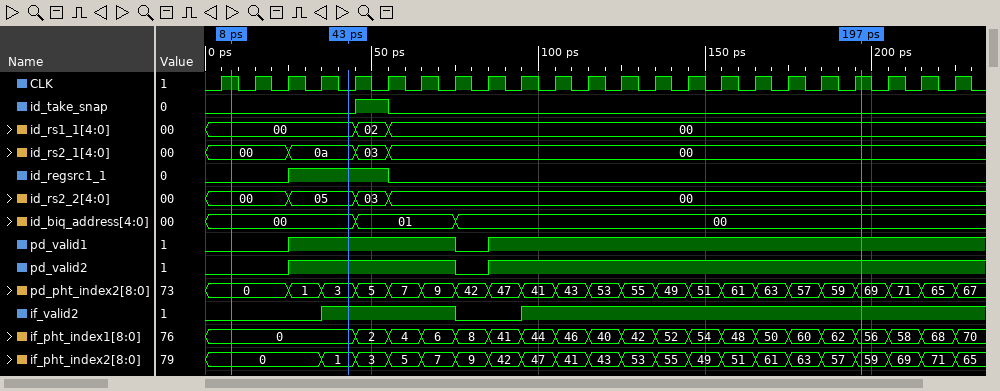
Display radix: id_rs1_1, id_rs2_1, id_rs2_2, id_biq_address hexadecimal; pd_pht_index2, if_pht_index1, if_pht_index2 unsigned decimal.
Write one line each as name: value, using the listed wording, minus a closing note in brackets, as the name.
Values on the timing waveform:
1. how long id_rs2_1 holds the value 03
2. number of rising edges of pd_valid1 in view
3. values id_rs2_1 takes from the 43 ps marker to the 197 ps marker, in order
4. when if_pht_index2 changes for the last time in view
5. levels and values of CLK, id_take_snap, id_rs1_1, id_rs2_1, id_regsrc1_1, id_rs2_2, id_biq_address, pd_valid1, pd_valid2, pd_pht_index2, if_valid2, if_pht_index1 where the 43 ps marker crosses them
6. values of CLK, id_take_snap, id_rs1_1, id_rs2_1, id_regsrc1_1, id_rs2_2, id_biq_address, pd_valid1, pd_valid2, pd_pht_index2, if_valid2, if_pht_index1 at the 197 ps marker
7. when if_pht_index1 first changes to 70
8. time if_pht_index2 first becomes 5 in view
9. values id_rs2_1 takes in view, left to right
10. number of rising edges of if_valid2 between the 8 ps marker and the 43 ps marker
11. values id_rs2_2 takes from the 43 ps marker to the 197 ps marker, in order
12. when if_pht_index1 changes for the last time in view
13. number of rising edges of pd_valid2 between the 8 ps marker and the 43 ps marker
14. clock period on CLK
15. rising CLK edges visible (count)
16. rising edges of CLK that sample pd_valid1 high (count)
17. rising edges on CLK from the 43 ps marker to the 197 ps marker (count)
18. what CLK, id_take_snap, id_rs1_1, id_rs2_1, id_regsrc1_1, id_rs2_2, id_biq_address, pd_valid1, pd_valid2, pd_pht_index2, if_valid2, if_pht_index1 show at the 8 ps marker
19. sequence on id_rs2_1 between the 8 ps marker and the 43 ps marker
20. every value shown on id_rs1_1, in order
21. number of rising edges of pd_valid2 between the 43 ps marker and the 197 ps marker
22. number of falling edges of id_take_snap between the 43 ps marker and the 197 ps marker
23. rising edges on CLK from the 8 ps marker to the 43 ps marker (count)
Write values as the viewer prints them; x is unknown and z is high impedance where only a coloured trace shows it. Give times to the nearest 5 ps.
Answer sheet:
how long id_rs2_1 holds the value 03: 10 ps
number of rising edges of pd_valid1 in view: 2
values id_rs2_1 takes from the 43 ps marker to the 197 ps marker, in order: 0a, 03, 00
when if_pht_index2 changes for the last time in view: 225 ps
levels and values of CLK, id_take_snap, id_rs1_1, id_rs2_1, id_regsrc1_1, id_rs2_2, id_biq_address, pd_valid1, pd_valid2, pd_pht_index2, if_valid2, if_pht_index1 where the 43 ps marker crosses them: CLK=0, id_take_snap=0, id_rs1_1=00, id_rs2_1=0a, id_regsrc1_1=1, id_rs2_2=05, id_biq_address=00, pd_valid1=1, pd_valid2=1, pd_pht_index2=3, if_valid2=1, if_pht_index1=0
values of CLK, id_take_snap, id_rs1_1, id_rs2_1, id_regsrc1_1, id_rs2_2, id_biq_address, pd_valid1, pd_valid2, pd_pht_index2, if_valid2, if_pht_index1 at the 197 ps marker: CLK=1, id_take_snap=0, id_rs1_1=00, id_rs2_1=00, id_regsrc1_1=0, id_rs2_2=00, id_biq_address=00, pd_valid1=1, pd_valid2=1, pd_pht_index2=69, if_valid2=1, if_pht_index1=56
when if_pht_index1 first changes to 70: 225 ps
time if_pht_index2 first becomes 5 in view: 55 ps
values id_rs2_1 takes in view, left to right: 00, 0a, 03, 00
number of rising edges of if_valid2 between the 8 ps marker and the 43 ps marker: 1
values id_rs2_2 takes from the 43 ps marker to the 197 ps marker, in order: 05, 03, 00
when if_pht_index1 changes for the last time in view: 225 ps
number of rising edges of pd_valid2 between the 8 ps marker and the 43 ps marker: 1
clock period on CLK: 10 ps
rising CLK edges visible: 23
rising edges of CLK that sample pd_valid1 high: 19
rising edges on CLK from the 43 ps marker to the 197 ps marker: 16
what CLK, id_take_snap, id_rs1_1, id_rs2_1, id_regsrc1_1, id_rs2_2, id_biq_address, pd_valid1, pd_valid2, pd_pht_index2, if_valid2, if_pht_index1 show at the 8 ps marker: CLK=1, id_take_snap=0, id_rs1_1=00, id_rs2_1=00, id_regsrc1_1=0, id_rs2_2=00, id_biq_address=00, pd_valid1=0, pd_valid2=0, pd_pht_index2=0, if_valid2=0, if_pht_index1=0
sequence on id_rs2_1 between the 8 ps marker and the 43 ps marker: 00, 0a
every value shown on id_rs1_1, in order: 00, 02, 00
number of rising edges of pd_valid2 between the 43 ps marker and the 197 ps marker: 1
number of falling edges of id_take_snap between the 43 ps marker and the 197 ps marker: 1
rising edges on CLK from the 8 ps marker to the 43 ps marker: 3
